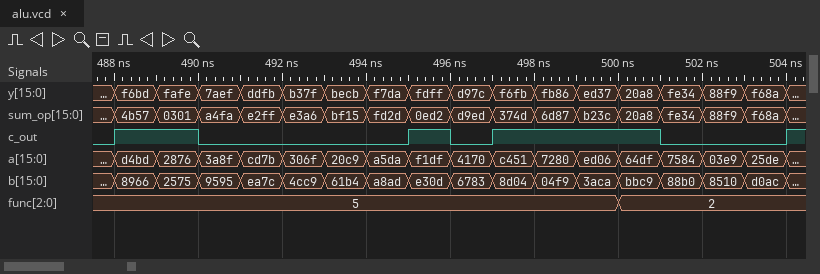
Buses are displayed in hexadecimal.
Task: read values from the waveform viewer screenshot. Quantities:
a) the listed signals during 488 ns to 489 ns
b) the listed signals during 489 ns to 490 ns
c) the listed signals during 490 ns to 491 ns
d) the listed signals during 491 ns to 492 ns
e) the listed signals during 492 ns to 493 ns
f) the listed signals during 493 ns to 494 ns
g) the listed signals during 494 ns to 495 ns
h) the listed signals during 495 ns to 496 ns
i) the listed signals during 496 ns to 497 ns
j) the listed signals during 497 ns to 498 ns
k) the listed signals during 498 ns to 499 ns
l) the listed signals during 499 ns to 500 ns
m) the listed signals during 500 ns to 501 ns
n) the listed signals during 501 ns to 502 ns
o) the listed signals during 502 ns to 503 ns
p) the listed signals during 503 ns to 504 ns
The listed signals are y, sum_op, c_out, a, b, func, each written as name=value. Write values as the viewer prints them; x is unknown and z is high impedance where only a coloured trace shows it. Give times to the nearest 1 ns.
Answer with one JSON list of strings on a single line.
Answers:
["y=f6bd, sum_op=4b57, c_out=1, a=d4bd, b=8966, func=5", "y=fafe, sum_op=0301, c_out=1, a=2876, b=2575, func=5", "y=7aef, sum_op=a4fa, c_out=0, a=3a8f, b=9595, func=5", "y=ddfb, sum_op=e2ff, c_out=0, a=cd7b, b=ea7c, func=5", "y=b37f, sum_op=e3a6, c_out=0, a=306f, b=4cc9, func=5", "y=becb, sum_op=bf15, c_out=0, a=20c9, b=61b4, func=5", "y=f7da, sum_op=fd2d, c_out=0, a=a5da, b=a8ad, func=5", "y=fdff, sum_op=0ed2, c_out=1, a=f1df, b=e30d, func=5", "y=d97c, sum_op=d9ed, c_out=0, a=4170, b=6783, func=5", "y=f6fb, sum_op=374d, c_out=1, a=c451, b=8d04, func=5", "y=fb86, sum_op=6d87, c_out=1, a=7280, b=04f9, func=5", "y=ed37, sum_op=b23c, c_out=1, a=ed06, b=3aca, func=5", "y=20a8, sum_op=20a8, c_out=1, a=64df, b=bbc9, func=2", "y=fe34, sum_op=fe34, c_out=0, a=7584, b=88b0, func=2", "y=88f9, sum_op=88f9, c_out=0, a=03e9, b=8510, func=2", "y=f68a, sum_op=f68a, c_out=0, a=25de, b=d0ac, func=2"]
